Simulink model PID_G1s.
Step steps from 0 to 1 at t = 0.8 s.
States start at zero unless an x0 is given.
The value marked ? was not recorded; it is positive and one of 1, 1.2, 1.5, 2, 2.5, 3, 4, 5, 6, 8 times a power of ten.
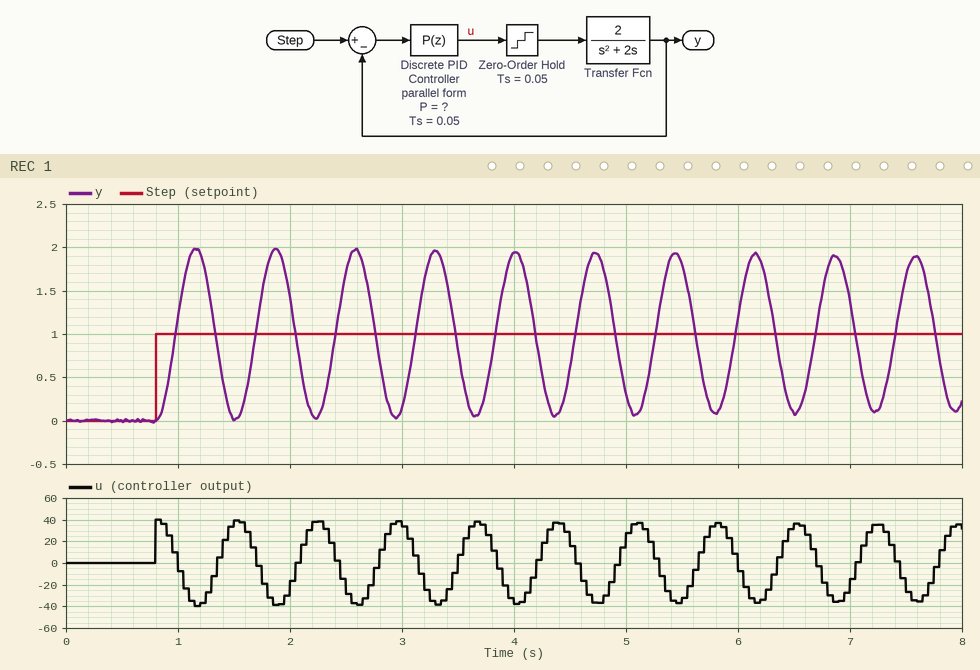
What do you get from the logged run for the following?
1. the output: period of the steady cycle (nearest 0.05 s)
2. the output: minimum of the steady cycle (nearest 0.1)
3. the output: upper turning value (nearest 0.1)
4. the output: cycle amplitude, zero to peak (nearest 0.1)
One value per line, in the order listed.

0.70 s
0.1
1.9
0.9
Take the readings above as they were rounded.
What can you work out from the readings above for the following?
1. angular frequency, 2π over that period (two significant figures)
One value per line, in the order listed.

9.0 rad/s
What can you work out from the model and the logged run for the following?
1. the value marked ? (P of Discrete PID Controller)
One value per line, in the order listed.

40
